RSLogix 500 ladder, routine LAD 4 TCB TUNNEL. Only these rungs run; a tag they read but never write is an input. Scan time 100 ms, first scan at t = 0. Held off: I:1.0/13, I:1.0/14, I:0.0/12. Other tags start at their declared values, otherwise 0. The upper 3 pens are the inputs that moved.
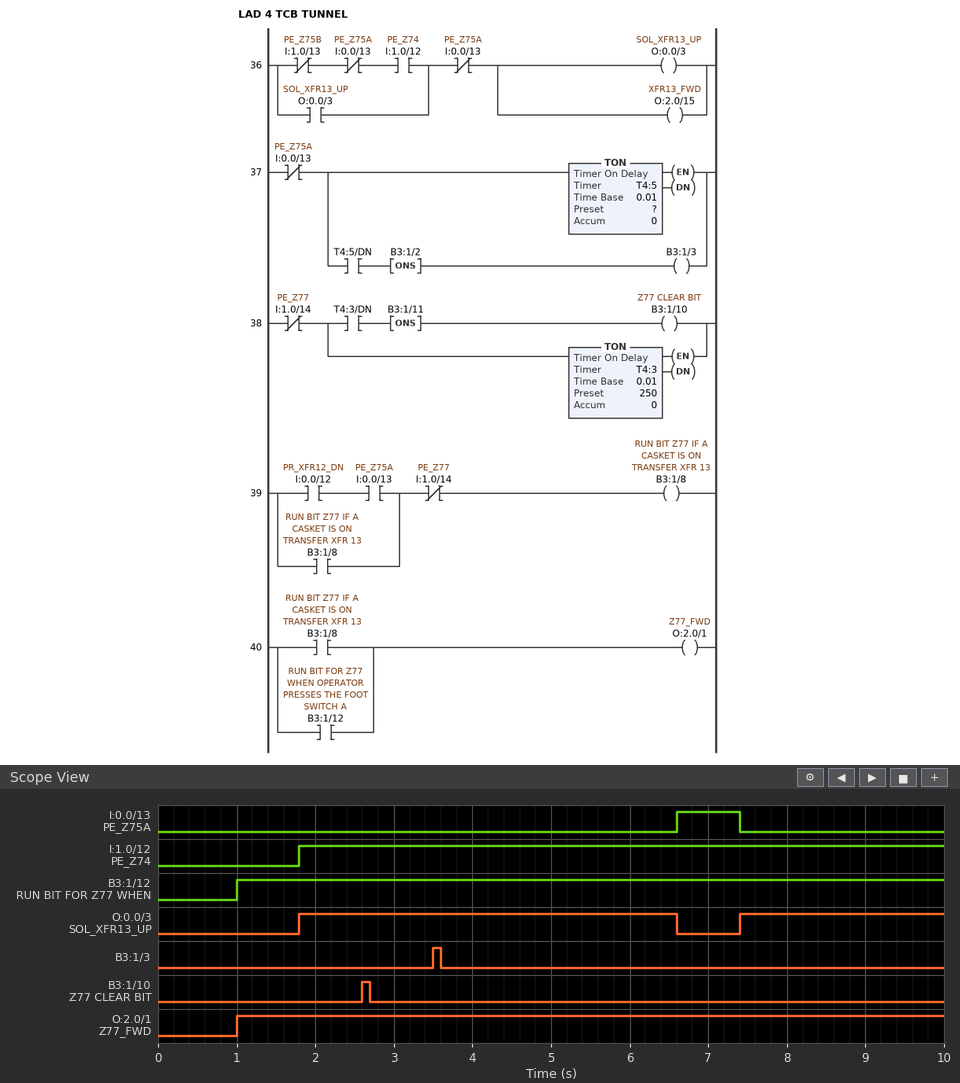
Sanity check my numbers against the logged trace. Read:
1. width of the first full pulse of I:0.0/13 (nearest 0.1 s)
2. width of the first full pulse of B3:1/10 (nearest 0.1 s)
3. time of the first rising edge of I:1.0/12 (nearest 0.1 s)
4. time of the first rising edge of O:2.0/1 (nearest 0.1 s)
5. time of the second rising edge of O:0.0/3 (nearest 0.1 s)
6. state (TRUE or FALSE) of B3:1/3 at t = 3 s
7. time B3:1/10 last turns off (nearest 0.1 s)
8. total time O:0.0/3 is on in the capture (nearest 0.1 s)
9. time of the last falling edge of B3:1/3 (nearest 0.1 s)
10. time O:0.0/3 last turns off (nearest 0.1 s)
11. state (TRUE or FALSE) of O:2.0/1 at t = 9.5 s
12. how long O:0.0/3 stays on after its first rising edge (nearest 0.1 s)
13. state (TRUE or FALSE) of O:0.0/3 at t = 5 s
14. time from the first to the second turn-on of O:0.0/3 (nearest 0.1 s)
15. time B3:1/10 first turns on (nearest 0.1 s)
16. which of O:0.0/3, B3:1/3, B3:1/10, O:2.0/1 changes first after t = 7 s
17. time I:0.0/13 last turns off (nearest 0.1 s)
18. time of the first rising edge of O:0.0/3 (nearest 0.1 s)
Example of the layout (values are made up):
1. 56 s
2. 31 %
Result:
1. 0.8 s
2. 0.1 s
3. 1.8 s
4. 1.0 s
5. 7.4 s
6. FALSE
7. 2.7 s
8. 7.4 s
9. 3.6 s
10. 6.6 s
11. TRUE
12. 4.8 s
13. TRUE
14. 5.6 s
15. 2.6 s
16. O:0.0/3
17. 7.4 s
18. 1.8 s
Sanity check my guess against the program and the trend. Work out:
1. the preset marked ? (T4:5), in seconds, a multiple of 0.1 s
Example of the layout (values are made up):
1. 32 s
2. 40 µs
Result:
1. 3.5 s
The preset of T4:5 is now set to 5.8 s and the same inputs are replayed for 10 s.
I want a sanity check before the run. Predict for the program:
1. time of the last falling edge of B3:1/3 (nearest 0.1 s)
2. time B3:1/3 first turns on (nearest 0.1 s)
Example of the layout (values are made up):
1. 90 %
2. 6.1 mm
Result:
1. 5.9 s
2. 5.8 s
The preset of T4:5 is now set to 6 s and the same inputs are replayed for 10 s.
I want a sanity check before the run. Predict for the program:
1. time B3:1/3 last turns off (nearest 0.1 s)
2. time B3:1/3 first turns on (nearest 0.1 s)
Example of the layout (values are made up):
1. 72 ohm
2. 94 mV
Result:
1. 6.1 s
2. 6.0 s
